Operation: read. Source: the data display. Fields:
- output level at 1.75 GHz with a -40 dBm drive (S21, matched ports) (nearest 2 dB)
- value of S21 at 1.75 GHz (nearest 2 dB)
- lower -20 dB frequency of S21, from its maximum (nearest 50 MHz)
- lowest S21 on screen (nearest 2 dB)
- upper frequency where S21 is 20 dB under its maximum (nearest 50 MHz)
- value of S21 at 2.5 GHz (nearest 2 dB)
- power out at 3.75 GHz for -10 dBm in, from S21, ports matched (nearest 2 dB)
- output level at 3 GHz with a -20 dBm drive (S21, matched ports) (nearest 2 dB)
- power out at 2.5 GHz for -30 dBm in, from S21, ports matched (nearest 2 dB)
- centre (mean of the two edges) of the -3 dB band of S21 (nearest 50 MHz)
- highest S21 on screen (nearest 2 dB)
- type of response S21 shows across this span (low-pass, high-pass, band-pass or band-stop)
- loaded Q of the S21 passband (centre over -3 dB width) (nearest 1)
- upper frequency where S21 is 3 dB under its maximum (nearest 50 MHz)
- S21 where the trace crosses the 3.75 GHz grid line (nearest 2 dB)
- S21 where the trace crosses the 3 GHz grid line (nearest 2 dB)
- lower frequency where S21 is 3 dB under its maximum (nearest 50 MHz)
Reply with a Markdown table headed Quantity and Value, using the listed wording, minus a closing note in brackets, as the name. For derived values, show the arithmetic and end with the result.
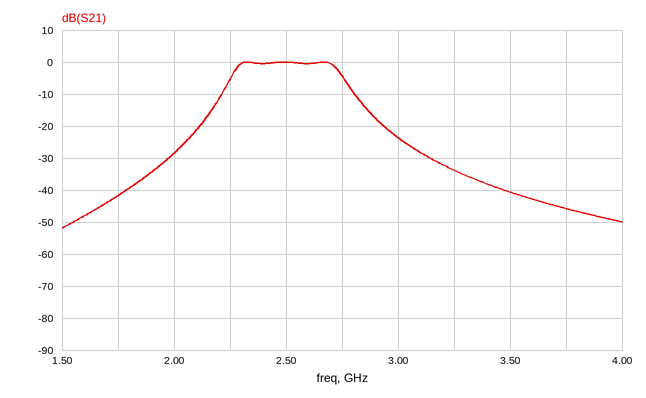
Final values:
| Quantity | Value |
|---|---|
| output level at 1.75 GHz with a -40 dBm drive (S21, matched ports) | -40 dBm + (-42 dB) = -82 dBm |
| value of S21 at 1.75 GHz | -42 dB |
| lower -20 dB frequency of S21, from its maximum | 2.10 GHz |
| lowest S21 on screen | -52 dB |
| upper frequency where S21 is 20 dB under its maximum | 2.95 GHz |
| value of S21 at 2.5 GHz | 0 dB |
| power out at 3.75 GHz for -10 dBm in, from S21, ports matched | -10 dBm + (-46 dB) = -56 dBm |
| output level at 3 GHz with a -20 dBm drive (S21, matched ports) | -20 dBm + (-24 dB) = -44 dBm |
| power out at 2.5 GHz for -30 dBm in, from S21, ports matched | -30 dBm + (0 dB) = -30 dBm |
| centre (mean of the two edges) of the -3 dB band of S21 | 2.50 GHz |
| highest S21 on screen | 0 dB |
| type of response S21 shows across this span | band-pass |
| loaded Q of the S21 passband (centre over -3 dB width) | 2.5 GHz / 500 MHz ≈ 5 |
| upper frequency where S21 is 3 dB under its maximum | 2.75 GHz |
| S21 where the trace crosses the 3.75 GHz grid line | -46 dB |
| S21 where the trace crosses the 3 GHz grid line | -24 dB |
| lower frequency where S21 is 3 dB under its maximum | 2.25 GHz |
